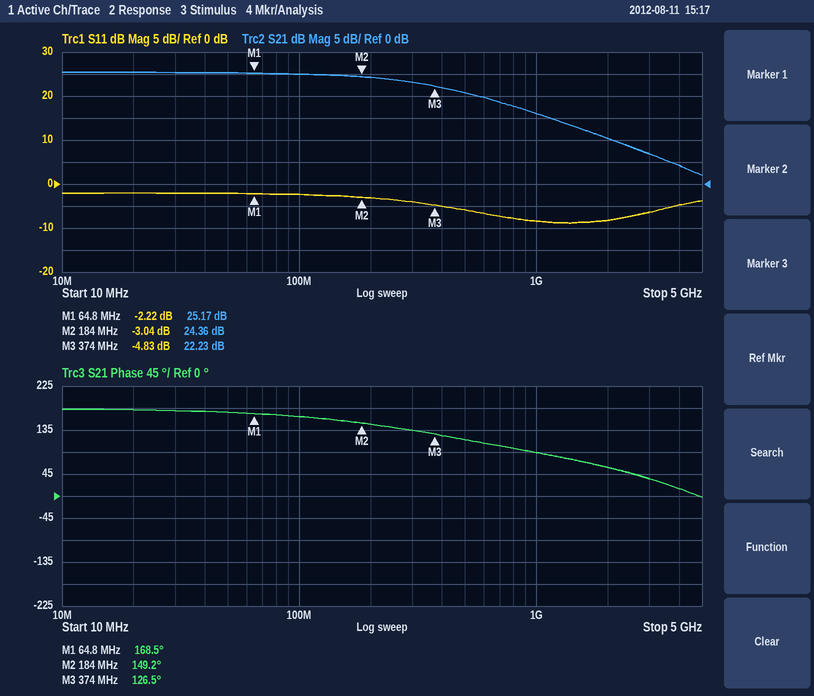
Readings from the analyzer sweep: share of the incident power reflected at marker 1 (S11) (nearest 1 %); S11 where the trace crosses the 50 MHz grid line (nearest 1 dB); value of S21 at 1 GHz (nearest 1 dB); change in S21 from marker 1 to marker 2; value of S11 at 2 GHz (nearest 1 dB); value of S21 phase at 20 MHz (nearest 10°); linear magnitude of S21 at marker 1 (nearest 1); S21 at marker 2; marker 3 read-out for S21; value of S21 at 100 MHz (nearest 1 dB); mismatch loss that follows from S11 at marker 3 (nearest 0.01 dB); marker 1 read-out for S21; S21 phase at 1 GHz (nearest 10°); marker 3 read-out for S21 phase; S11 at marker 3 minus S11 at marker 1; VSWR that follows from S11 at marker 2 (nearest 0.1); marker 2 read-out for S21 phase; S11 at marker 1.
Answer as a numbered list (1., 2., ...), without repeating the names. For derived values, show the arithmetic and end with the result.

1. 10^(-2.22/10) ≈ 60 %
2. -2 dB
3. 16 dB
4. 24.36 − (25.17) = -0.81 dB
5. -8 dB
6. 180°
7. 10^(25.17/20) ≈ 18
8. 24.36 dB
9. 22.23 dB
10. 25 dB
11. −10 log10(1 − 10^(-4.83/10)) ≈ 1.73 dB
12. 25.17 dB
13. 90°
14. 126.5°
15. -4.83 − (-2.22) = -2.61 dB
16. (1 + 0.7047)/(1 − 0.7047) ≈ 5.8
17. 149.2°
18. -2.22 dB
